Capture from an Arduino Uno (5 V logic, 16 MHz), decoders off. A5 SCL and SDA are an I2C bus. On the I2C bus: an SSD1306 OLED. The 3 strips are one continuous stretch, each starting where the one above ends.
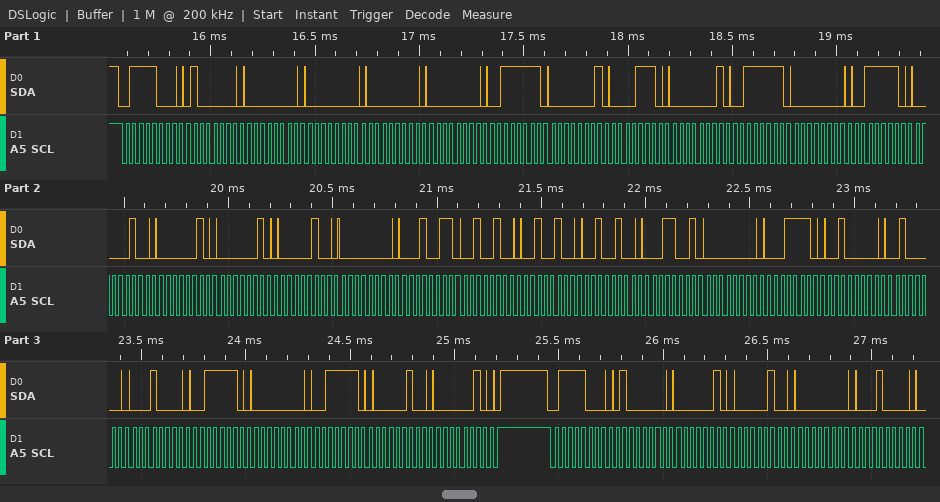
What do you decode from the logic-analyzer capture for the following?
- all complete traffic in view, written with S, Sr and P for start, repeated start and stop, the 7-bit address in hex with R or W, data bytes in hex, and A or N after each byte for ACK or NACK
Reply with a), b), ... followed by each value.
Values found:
a) S 3CW A 40 A 00 A 00 A 00 A 00 A 3F A 01 A 0E A 01 A 3F A 00 A 3E A 04 A 02 A 02 A 04 A 00 A 13 A 24 A 24 A 24 A 19 A 00 A 1E A 20 A 20 A 10 A 3E A 00 A 3E A 04 A 02 A P S 3CW A 40 A 02 A 04 A 00 A 10 A
